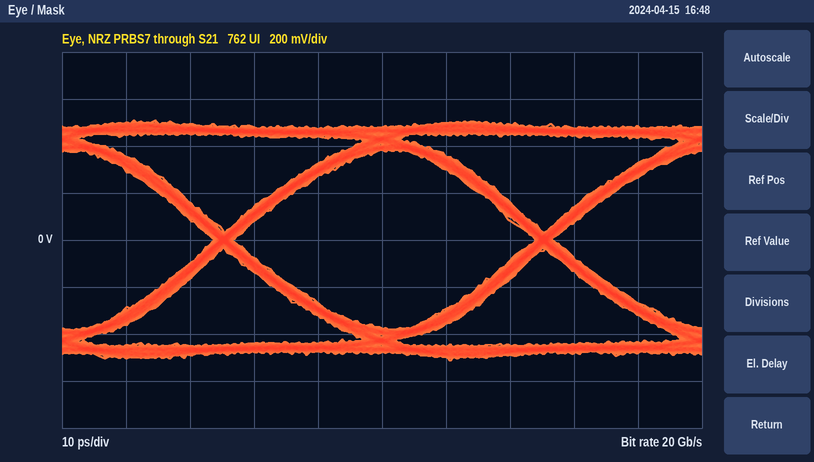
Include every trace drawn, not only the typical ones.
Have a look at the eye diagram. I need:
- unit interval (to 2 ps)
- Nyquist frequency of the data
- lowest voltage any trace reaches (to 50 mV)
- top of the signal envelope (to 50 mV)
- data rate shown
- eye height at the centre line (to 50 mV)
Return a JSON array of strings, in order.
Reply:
["50 ps", "10 GHz", "-500 mV", "500 mV", "20 Gb/s", "750 mV"]
